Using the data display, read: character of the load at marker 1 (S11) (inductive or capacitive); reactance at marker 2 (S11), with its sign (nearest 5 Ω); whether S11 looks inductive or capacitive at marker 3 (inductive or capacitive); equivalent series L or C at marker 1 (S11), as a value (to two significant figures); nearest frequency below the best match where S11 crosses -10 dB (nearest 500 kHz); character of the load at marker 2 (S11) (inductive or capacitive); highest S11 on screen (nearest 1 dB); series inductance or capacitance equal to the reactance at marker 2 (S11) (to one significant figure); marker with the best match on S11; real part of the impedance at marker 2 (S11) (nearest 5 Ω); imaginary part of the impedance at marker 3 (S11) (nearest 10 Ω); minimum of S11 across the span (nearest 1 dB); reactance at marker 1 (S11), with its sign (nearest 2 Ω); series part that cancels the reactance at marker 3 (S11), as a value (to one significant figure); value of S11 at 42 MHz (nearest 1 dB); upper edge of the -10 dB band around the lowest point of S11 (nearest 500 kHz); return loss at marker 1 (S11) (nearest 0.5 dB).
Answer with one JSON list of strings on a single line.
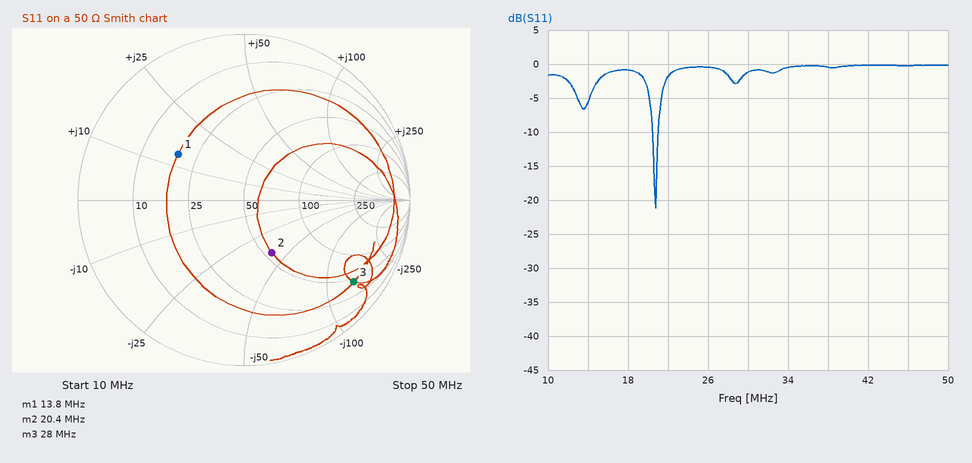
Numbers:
["inductive", "-40 Ω", "capacitive", "160 nH", "20.5 MHz", "capacitive", "0 dB", "200 pF", "marker 2", "55 Ω", "-140 Ω", "-21 dB", "+14 Ω", "800 nH", "0 dB", "21.0 MHz", "6.5 dB"]
